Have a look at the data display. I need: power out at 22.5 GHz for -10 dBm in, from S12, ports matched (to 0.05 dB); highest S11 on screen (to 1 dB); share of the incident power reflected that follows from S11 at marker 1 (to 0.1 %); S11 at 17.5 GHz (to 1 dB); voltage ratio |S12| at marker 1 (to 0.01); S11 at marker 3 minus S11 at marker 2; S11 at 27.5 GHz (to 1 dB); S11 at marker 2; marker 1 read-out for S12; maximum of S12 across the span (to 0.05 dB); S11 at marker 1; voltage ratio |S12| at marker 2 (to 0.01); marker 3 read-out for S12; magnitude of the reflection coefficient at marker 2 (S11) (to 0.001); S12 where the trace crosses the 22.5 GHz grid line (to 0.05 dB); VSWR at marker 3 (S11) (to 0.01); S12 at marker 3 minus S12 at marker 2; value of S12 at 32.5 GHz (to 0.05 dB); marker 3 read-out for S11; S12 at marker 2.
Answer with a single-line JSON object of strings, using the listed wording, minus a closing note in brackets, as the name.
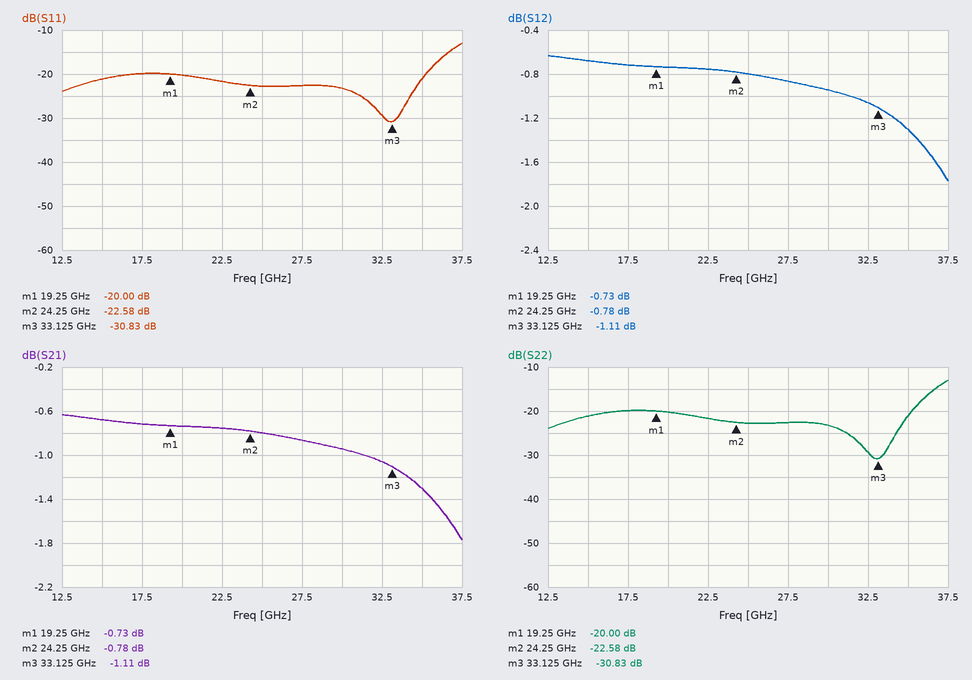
{"power out at 22.5 GHz for -10 dBm in, from S12, ports matched": "-10.75 dBm", "highest S11 on screen": "-13 dB", "share of the incident power reflected that follows from S11 at marker 1": "1.0 %", "S11 at 17.5 GHz": "-20 dB", "voltage ratio |S12| at marker 1": "0.92", "S11 at marker 3 minus S11 at marker 2": "-8.25 dB", "S11 at 27.5 GHz": "-23 dB", "S11 at marker 2": "-22.58 dB", "marker 1 read-out for S12": "-0.73 dB", "maximum of S12 across the span": "-0.65 dB", "S11 at marker 1": "-20.00 dB", "voltage ratio |S12| at marker 2": "0.91", "marker 3 read-out for S12": "-1.11 dB", "magnitude of the reflection coefficient at marker 2 (S11)": "0.074", "S12 where the trace crosses the 22.5 GHz grid line": "-0.75 dB", "VSWR at marker 3 (S11)": "1.06", "S12 at marker 3 minus S12 at marker 2": "-0.33 dB", "value of S12 at 32.5 GHz": "-1.05 dB", "marker 3 read-out for S11": "-30.83 dB", "S12 at marker 2": "-0.78 dB"}
